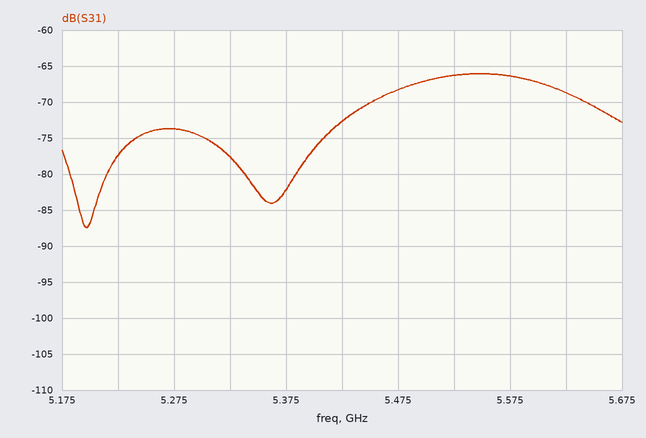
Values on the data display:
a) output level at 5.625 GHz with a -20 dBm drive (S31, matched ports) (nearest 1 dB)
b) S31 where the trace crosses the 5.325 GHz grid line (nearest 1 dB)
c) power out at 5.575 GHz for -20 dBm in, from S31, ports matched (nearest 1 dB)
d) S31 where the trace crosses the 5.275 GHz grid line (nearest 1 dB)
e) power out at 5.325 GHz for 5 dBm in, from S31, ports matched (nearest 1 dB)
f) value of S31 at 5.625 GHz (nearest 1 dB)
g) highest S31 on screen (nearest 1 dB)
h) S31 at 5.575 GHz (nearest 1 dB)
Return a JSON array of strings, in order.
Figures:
["-89 dBm", "-78 dB", "-86 dBm", "-74 dB", "-73 dBm", "-69 dB", "-66 dB", "-66 dB"]
